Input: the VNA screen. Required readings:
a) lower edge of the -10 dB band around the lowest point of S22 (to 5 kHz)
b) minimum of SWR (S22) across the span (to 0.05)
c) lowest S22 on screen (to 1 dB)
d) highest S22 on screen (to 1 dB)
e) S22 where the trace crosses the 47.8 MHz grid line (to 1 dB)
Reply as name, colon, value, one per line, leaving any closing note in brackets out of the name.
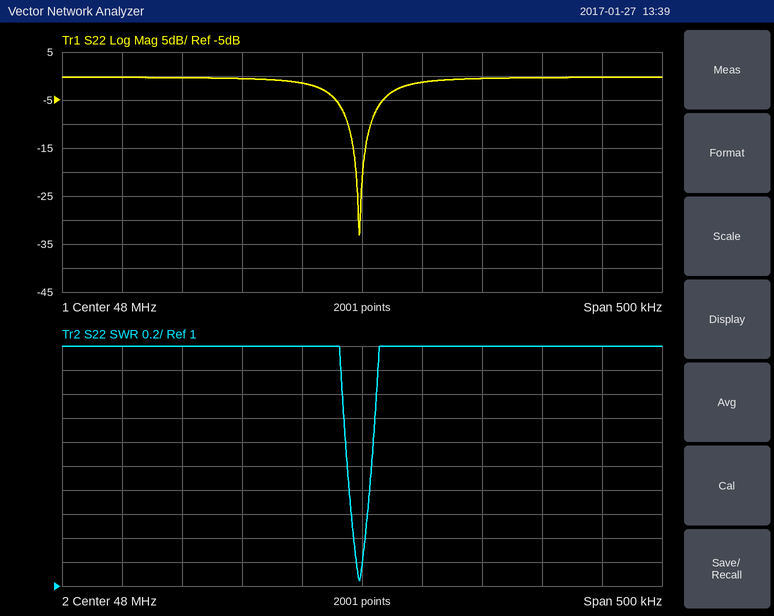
lower edge of the -10 dB band around the lowest point of S22: 47.990 MHz
minimum of SWR (S22) across the span: 1.05
lowest S22 on screen: -33 dB
highest S22 on screen: 0 dB
S22 where the trace crosses the 47.8 MHz grid line: 0 dB
